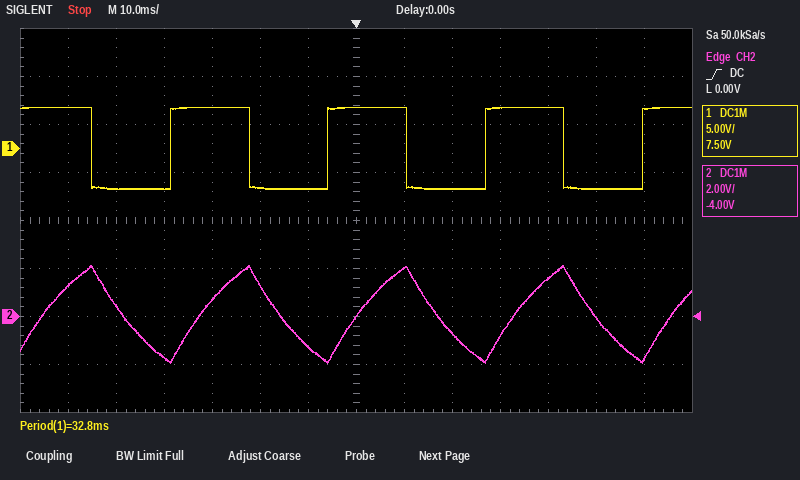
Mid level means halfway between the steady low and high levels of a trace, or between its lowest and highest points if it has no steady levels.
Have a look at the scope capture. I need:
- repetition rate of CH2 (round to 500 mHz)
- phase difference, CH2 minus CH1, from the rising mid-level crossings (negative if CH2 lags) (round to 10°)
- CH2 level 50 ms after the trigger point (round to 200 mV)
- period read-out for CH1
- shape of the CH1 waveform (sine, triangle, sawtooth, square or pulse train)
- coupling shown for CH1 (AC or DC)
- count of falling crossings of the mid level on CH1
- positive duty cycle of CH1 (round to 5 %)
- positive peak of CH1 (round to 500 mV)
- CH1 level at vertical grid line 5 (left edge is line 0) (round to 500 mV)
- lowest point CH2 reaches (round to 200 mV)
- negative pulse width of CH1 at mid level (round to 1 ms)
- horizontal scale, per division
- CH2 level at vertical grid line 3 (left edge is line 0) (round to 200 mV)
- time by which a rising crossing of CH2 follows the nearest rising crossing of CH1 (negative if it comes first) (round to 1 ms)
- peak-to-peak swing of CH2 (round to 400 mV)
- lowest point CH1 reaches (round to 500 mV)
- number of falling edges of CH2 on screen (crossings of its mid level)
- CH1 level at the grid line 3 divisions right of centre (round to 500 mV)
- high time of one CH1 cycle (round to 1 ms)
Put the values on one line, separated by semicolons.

30.5 Hz; -70°; 0.0 V; 32.8 ms; square; DC; 4; 50 %; 4.5 V; -4.0 V; -2.0 V; 16 ms; 10 ms; -1.8 V; +6 ms; 4.0 V; -4.5 V; 4; 4.0 V; 16 ms
